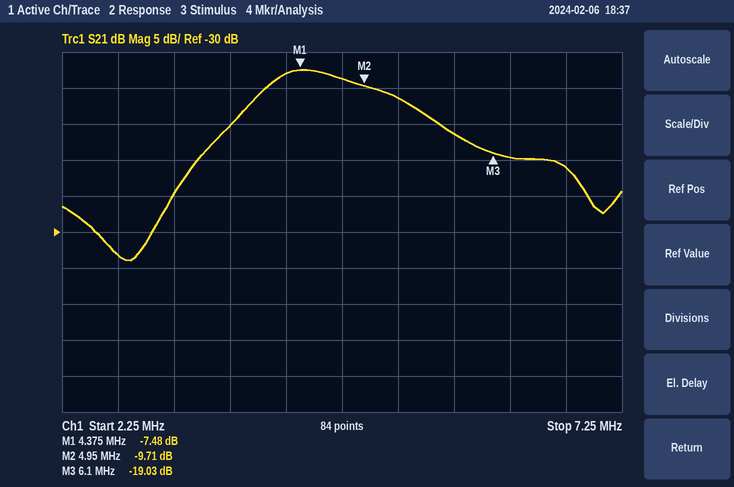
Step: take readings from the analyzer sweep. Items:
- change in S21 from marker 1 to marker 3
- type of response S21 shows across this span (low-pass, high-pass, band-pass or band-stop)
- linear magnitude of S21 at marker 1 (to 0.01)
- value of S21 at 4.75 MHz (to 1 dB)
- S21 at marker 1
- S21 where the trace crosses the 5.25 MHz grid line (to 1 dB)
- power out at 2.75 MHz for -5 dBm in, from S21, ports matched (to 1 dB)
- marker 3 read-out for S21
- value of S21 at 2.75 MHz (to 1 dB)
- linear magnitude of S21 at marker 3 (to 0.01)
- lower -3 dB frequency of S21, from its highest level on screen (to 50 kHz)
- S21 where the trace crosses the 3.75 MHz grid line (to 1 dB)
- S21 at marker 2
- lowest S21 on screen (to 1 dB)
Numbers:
-11.55 dB
band-pass
0.42
-9 dB
-7.48 dB
-11 dB
-38 dBm
-19.03 dB
-33 dB
0.11
4.05 MHz
-15 dB
-9.71 dB
-34 dB
